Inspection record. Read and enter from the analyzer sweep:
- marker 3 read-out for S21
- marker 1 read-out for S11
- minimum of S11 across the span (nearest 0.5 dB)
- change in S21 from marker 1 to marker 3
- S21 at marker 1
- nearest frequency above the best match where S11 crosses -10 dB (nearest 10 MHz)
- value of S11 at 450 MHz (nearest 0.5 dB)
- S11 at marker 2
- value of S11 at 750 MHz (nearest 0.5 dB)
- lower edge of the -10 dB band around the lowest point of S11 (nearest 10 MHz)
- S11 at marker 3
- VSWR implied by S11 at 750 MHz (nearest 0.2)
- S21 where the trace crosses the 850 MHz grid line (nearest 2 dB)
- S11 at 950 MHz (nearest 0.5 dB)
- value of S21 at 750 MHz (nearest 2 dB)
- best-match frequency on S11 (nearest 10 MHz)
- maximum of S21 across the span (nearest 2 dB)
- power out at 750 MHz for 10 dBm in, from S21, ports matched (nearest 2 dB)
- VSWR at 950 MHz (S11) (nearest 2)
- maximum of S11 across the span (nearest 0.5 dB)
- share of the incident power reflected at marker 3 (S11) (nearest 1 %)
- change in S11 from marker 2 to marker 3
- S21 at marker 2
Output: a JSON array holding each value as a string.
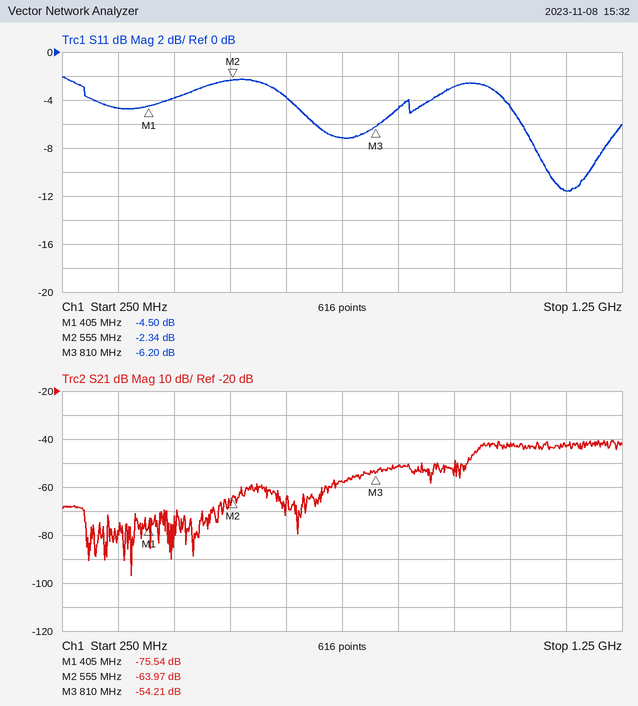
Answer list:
["-54.21 dB", "-4.50 dB", "-11.5 dB", "21.33 dB", "-75.54 dB", "1.19 GHz", "-4.0 dB", "-2.34 dB", "-7.0 dB", "1.12 GHz", "-6.20 dB", "2.6", "-52 dB", "-3.0 dB", "-58 dB", "1.15 GHz", "-40 dB", "-48 dBm", "6", "-2.0 dB", "24 %", "-3.86 dB", "-63.97 dB"]
